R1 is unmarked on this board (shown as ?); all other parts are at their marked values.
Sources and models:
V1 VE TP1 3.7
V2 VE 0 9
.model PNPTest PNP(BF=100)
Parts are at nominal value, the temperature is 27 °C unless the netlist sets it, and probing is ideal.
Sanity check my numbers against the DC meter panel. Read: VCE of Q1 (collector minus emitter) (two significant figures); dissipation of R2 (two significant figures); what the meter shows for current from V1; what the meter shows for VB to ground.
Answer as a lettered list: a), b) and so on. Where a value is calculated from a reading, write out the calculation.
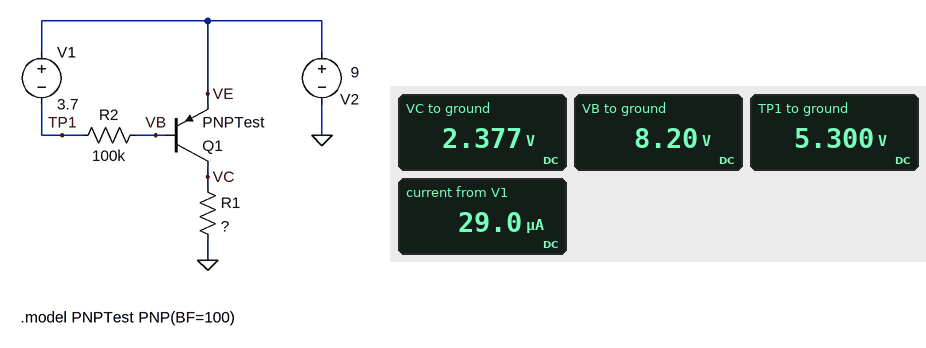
a) 2.377 V - 9 V = -6.6 V
b) (8.2 V - 5.3 V)^2 / 100 kΩ = 84 µW
c) 29.0 µA
d) 8.20 V
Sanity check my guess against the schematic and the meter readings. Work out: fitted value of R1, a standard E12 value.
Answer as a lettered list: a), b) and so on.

a) 820 Ω
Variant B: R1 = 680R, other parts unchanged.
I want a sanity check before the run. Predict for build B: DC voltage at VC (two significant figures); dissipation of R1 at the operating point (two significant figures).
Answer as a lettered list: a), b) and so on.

a) 2.0 V
b) 5.7 mW
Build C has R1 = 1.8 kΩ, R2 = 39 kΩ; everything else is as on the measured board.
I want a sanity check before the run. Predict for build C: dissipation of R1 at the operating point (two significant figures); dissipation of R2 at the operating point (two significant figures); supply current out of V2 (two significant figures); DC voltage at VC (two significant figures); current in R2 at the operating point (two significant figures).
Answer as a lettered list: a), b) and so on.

a) 44 mW
b) 210 µW
c) 4.9 mA
d) 8.9 V
e) 74 µA
